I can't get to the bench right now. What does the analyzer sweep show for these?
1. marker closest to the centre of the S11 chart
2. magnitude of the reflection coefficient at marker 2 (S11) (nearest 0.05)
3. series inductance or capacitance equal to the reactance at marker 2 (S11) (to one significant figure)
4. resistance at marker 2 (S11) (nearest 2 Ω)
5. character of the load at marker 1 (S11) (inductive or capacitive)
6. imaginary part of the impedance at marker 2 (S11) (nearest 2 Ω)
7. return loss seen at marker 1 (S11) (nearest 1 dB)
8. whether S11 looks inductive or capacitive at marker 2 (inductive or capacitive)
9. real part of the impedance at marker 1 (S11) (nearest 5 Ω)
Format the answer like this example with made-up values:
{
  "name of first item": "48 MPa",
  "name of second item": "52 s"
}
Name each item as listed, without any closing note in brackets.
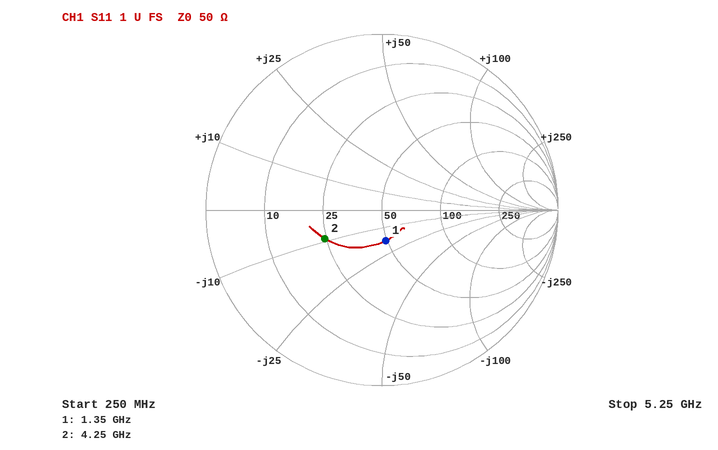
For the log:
{
  "marker closest to the centre of the S11 chart": "marker 1",
  "magnitude of the reflection coefficient at marker 2 (S11)": "0.35",
  "series inductance or capacitance equal to the reactance at marker 2 (S11)": "4 pF",
  "resistance at marker 2 (S11)": "24 Ω",
  "character of the load at marker 1 (S11)": "capacitive",
  "imaginary part of the impedance at marker 2 (S11)": "-10 Ω",
  "return loss seen at marker 1 (S11)": "15 dB",
  "whether S11 looks inductive or capacitive at marker 2": "capacitive",
  "real part of the impedance at marker 1 (S11)": "50 Ω"
}
